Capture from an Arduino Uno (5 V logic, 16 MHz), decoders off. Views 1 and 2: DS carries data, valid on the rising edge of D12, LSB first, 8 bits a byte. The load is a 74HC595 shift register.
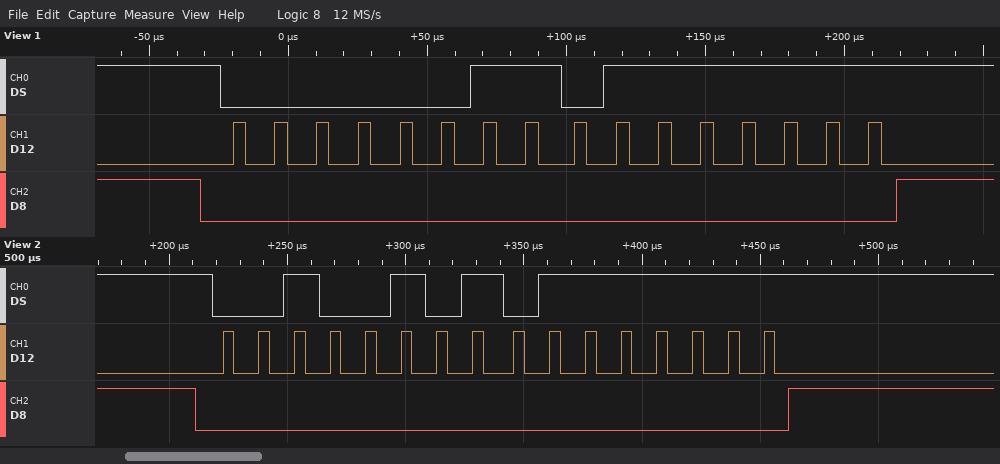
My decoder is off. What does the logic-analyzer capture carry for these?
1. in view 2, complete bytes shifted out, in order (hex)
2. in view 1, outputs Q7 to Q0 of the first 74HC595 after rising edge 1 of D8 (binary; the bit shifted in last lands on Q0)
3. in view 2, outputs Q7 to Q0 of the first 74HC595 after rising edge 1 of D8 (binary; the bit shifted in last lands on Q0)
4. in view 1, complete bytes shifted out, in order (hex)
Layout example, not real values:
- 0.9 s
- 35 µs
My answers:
- A4 FE
- 01111111
- 01111111
- 0xC0 0xFE
